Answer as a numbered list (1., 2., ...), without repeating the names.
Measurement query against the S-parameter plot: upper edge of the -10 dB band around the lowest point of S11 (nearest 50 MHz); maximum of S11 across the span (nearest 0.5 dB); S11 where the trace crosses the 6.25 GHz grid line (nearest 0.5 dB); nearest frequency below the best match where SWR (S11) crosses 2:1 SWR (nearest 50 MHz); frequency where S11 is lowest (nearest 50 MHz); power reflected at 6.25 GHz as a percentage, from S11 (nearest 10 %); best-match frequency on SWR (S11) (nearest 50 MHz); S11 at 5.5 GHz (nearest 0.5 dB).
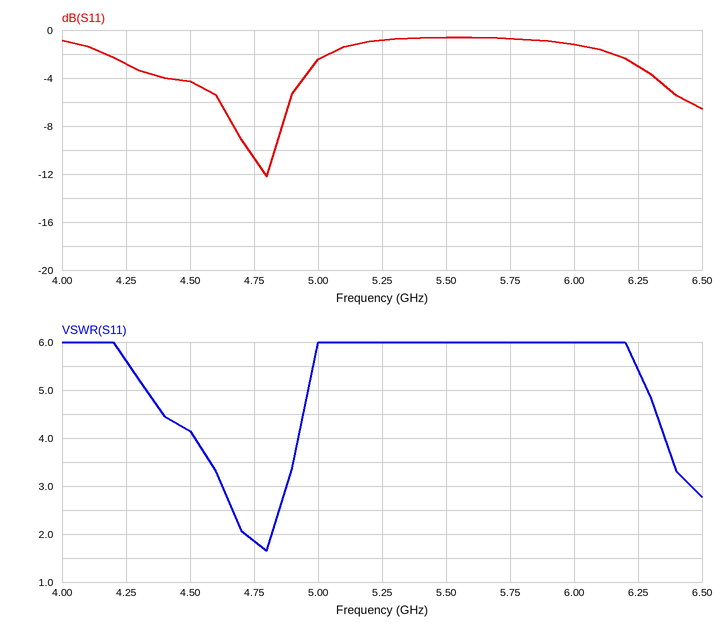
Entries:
1. 4.85 GHz
2. -0.5 dB
3. -3.0 dB
4. 4.70 GHz
5. 4.80 GHz
6. 50 %
7. 4.80 GHz
8. -0.5 dB
